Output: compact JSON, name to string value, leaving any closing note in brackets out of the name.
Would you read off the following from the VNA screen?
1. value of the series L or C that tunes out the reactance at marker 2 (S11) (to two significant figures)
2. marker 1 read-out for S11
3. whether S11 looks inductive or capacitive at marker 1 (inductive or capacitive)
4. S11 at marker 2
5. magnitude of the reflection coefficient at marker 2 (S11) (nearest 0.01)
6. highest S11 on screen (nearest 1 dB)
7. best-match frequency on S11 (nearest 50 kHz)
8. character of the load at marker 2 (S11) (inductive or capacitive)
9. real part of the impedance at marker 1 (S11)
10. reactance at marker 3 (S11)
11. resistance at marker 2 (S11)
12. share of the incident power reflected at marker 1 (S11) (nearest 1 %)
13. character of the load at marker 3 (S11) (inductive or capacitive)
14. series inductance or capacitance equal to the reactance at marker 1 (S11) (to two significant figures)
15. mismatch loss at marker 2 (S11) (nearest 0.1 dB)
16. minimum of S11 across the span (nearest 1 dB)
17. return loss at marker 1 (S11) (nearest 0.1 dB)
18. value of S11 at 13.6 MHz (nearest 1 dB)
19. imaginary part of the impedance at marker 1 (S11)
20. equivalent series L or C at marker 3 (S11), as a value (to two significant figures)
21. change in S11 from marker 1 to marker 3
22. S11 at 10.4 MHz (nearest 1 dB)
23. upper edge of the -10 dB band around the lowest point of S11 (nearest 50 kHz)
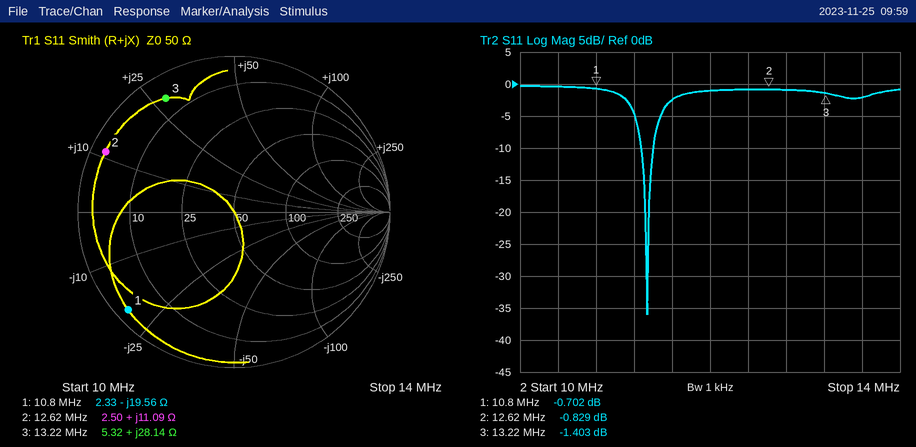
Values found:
{"value of the series L or C that tunes out the reactance at marker 2 (S11)": "1.1 nF", "marker 1 read-out for S11": "-0.702 dB", "whether S11 looks inductive or capacitive at marker 1": "capacitive", "S11 at marker 2": "-0.829 dB", "magnitude of the reflection coefficient at marker 2 (S11)": "0.91", "highest S11 on screen": "0 dB", "best-match frequency on S11": "11.35 MHz", "character of the load at marker 2 (S11)": "inductive", "real part of the impedance at marker 1": "2.33 Ω", "reactance at marker 3": "+28.14 Ω", "resistance at marker 2": "2.50 Ω", "share of the incident power reflected at marker 1 (S11)": "85 %", "character of the load at marker 3 (S11)": "inductive", "series inductance or capacitance equal to the reactance at marker 1 (S11)": "750 pF", "mismatch loss at marker 2 (S11)": "7.6 dB", "minimum of S11 across the span": "-36 dB", "return loss at marker 1 (S11)": "0.7 dB", "value of S11 at 13.6 MHz": "-2 dB", "imaginary part of the impedance at marker 1": "-19.56 Ω", "equivalent series L or C at marker 3 (S11), as a value": "340 nH", "change in S11 from marker 1 to marker 3": "-0.701 dB", "S11 at 10.4 MHz": "0 dB", "upper edge of the -10 dB band around the lowest point of S11": "11.40 MHz"}
